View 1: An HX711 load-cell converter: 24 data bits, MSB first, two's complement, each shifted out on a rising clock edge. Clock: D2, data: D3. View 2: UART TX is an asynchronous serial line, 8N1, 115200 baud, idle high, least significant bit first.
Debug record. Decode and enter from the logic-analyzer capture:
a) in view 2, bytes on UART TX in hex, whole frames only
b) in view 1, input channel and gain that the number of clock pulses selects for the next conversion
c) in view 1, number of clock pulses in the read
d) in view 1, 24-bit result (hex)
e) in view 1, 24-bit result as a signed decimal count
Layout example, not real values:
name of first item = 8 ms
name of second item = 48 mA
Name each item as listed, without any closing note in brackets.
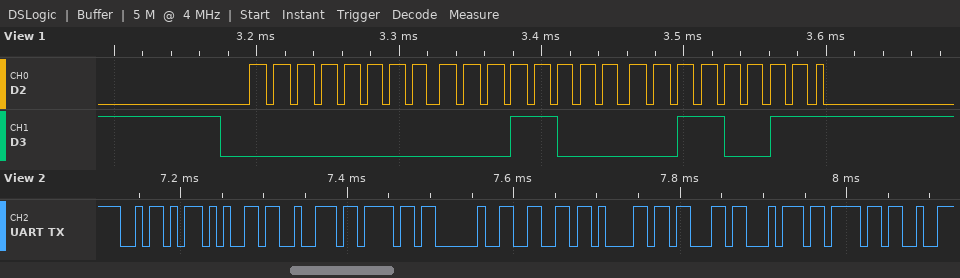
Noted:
in view 2, bytes on UART TX in hex, whole frames only = 5A 65 72 6F 20 66 61 63 74 6F
in view 1, input channel and gain that the number of clock pulses selects for the next conversion = channel A, gain 128
in view 1, number of clock pulses in the read = 25
in view 1, 24-bit result = 0x001833
in view 1, 24-bit result as a signed decimal count = 6195
